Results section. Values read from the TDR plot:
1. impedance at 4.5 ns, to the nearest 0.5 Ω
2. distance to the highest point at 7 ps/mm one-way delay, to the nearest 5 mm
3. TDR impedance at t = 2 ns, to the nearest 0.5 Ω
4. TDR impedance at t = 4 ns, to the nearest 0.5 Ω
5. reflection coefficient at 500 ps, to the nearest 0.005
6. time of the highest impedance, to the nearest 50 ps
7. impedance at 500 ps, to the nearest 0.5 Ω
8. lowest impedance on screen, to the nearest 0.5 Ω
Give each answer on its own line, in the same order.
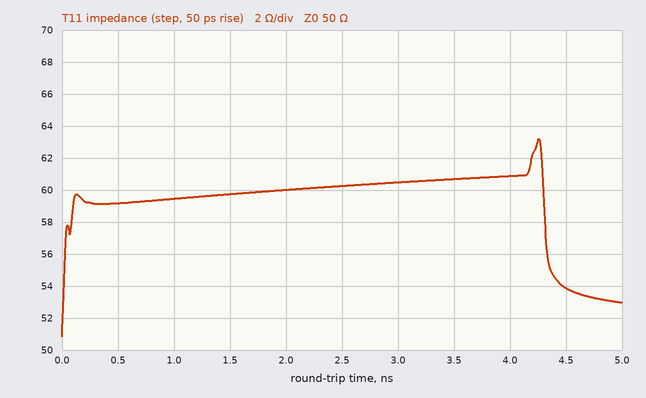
54.0 Ω
305 mm
60.0 Ω
61.0 Ω
+0.085
4.25 ns
59.0 Ω
51.0 Ω
